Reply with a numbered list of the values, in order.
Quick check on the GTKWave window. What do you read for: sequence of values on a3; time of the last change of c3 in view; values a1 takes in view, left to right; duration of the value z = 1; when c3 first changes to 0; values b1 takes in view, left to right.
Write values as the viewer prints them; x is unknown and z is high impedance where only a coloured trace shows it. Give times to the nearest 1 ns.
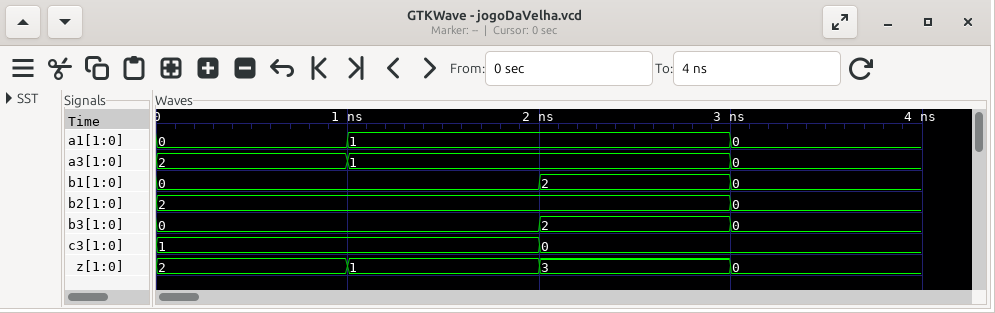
1. 2, 1, 0
2. 2 ns
3. 0, 1, 0
4. 1 ns
5. 2 ns
6. 0, 2, 0
